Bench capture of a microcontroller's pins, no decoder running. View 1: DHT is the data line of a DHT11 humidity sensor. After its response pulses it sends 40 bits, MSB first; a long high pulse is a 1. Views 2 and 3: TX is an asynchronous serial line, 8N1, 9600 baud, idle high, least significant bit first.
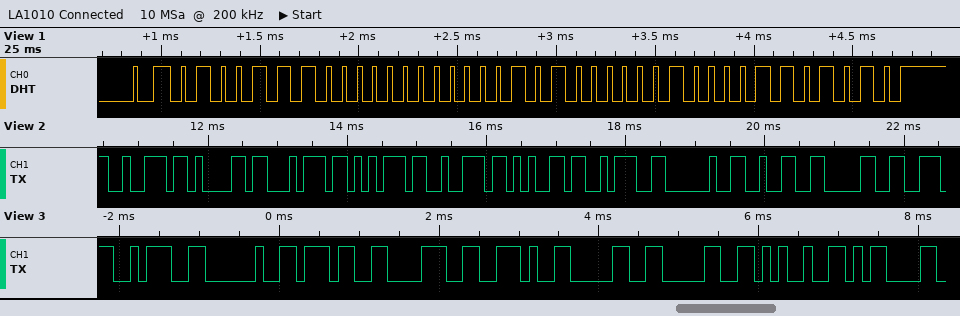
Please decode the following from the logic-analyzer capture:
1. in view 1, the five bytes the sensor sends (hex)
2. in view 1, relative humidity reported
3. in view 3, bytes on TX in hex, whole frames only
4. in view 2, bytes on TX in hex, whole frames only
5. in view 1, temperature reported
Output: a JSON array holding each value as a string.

["4E 00 14 08 6A", "78 %", "3A 20 37 38 2E 30 30 25 0D", "72 61 74 75 72 65 3A 20 32 30", "20.8 °C"]
